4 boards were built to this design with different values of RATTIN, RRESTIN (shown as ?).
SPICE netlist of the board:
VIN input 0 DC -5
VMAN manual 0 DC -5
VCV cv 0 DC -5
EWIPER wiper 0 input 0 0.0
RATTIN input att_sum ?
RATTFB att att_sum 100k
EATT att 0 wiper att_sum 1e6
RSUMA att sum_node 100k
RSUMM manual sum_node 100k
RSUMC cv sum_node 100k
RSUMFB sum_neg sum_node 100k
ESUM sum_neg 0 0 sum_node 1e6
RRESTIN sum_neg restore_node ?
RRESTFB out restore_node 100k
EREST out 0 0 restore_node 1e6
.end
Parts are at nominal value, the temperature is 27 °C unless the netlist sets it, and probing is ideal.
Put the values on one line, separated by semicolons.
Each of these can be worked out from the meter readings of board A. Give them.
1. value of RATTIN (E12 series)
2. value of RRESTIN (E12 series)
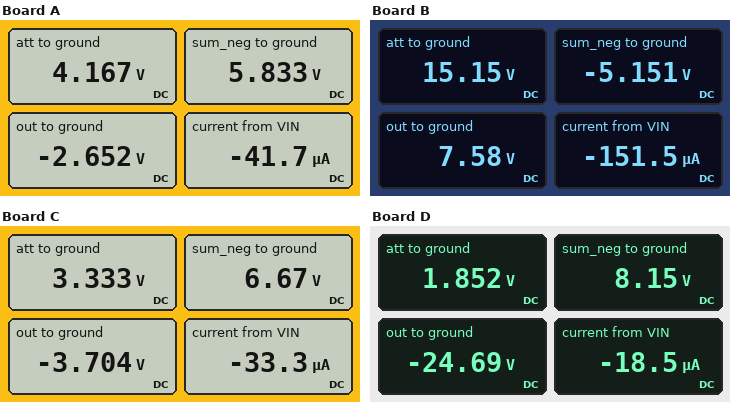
120 kΩ; 220 kΩ
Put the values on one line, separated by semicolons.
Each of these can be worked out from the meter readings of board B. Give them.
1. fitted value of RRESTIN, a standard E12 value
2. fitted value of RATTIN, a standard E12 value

68 kΩ; 33 kΩ
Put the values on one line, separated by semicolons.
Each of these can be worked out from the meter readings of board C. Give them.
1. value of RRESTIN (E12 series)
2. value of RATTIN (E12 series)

180 kΩ; 150 kΩ
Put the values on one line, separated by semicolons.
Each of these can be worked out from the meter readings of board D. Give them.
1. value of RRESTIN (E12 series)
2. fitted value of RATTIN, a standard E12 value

33 kΩ; 270 kΩ
